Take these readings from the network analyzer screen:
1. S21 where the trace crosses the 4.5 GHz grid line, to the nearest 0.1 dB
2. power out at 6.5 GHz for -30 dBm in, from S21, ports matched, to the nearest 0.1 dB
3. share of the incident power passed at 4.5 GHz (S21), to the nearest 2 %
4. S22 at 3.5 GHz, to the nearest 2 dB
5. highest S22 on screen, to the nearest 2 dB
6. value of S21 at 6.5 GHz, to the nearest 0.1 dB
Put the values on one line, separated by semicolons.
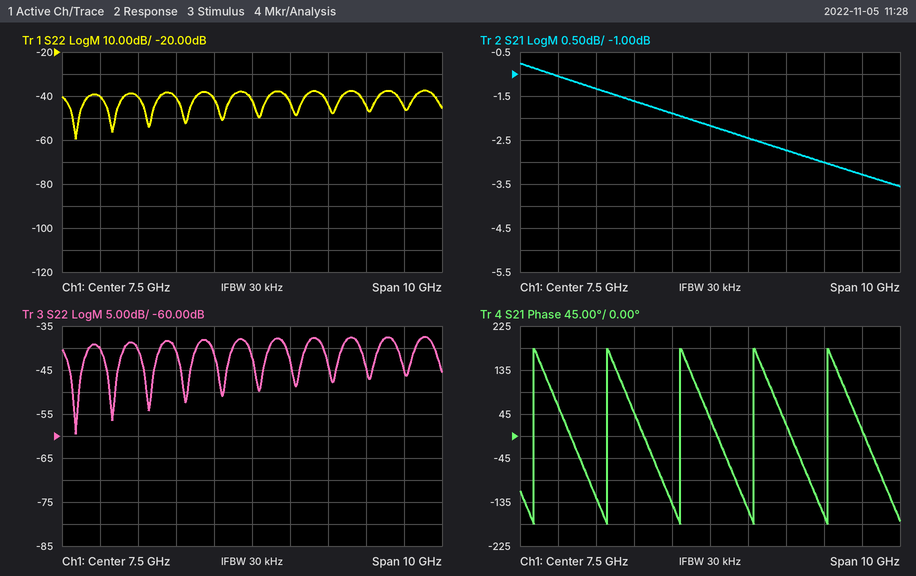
-1.3 dB; -31.9 dBm; 74 %; -40 dB; -38 dB; -1.9 dB
